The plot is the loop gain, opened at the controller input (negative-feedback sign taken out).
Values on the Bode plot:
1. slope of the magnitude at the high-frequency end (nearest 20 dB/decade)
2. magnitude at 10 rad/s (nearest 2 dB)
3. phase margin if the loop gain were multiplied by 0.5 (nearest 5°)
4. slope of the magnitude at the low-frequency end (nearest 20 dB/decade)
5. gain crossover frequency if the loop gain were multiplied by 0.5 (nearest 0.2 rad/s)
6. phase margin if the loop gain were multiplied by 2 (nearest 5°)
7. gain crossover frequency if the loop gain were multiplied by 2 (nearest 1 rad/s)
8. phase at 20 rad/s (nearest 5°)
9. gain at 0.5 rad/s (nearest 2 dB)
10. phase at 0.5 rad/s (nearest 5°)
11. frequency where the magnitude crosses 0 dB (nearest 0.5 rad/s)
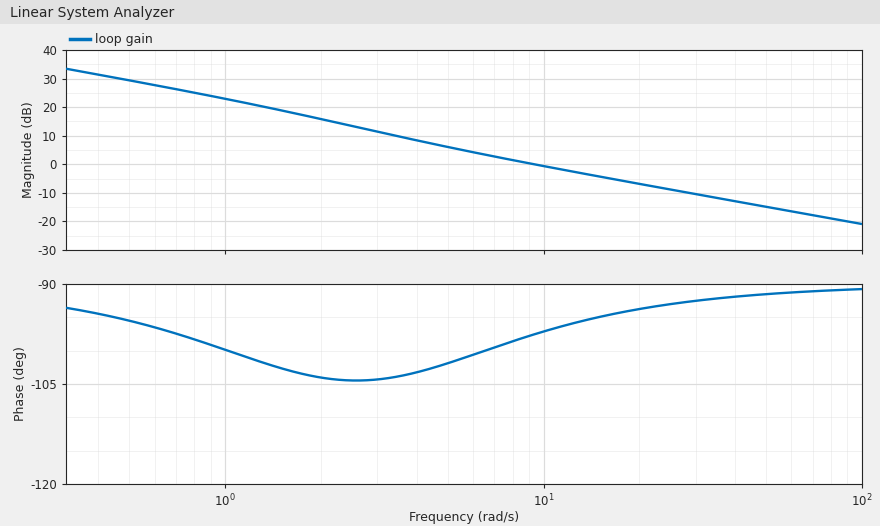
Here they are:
-20 dB/decade
0 dB
80°
-20 dB/decade
5.0 rad/s
85°
18 rad/s
-95°
30 dB
-95°
9.5 rad/s
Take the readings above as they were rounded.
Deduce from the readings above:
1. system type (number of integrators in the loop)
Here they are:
1
